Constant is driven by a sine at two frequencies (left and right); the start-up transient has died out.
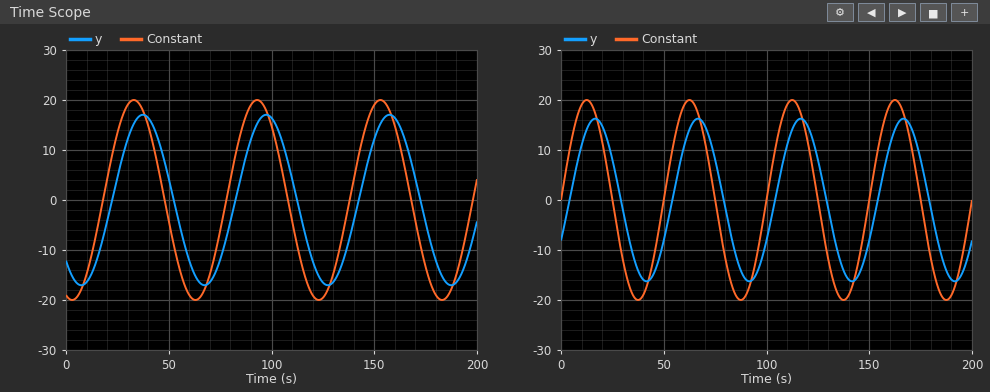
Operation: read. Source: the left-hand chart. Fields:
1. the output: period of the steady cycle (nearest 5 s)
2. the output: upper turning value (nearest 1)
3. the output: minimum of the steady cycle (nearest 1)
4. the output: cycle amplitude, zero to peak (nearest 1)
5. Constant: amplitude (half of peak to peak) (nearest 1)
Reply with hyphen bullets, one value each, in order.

- 60 s
- 17
- -17
- 17
- 20
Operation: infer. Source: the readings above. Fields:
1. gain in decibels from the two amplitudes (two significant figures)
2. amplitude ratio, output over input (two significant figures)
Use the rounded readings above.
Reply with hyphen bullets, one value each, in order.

- -1.4 dB
- 0.85
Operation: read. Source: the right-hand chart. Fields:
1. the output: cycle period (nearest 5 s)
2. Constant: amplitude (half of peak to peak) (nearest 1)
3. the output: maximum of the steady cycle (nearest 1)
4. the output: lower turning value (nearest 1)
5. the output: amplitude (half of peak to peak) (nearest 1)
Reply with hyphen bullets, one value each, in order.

- 50 s
- 20
- 16
- -16
- 16
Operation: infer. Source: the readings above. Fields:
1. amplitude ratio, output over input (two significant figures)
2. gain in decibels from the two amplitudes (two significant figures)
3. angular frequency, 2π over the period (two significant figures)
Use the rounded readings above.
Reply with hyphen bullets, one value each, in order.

- 0.80
- -1.9 dB
- 0.13 rad/s
